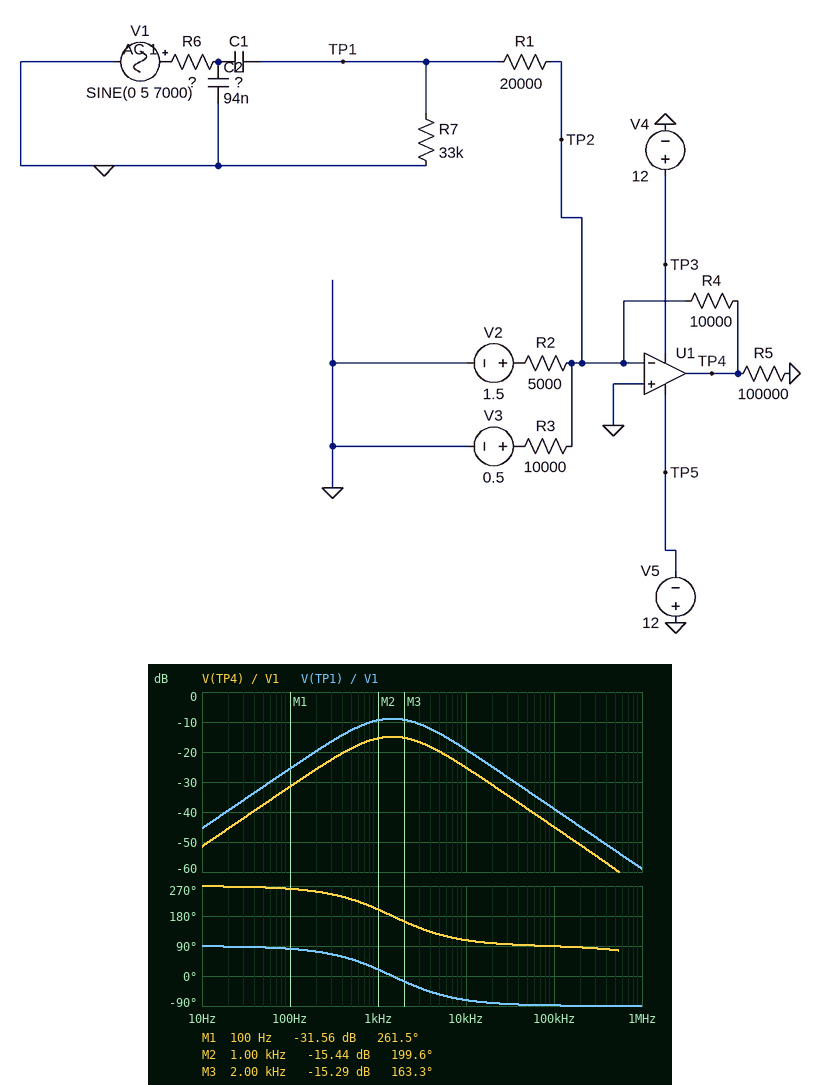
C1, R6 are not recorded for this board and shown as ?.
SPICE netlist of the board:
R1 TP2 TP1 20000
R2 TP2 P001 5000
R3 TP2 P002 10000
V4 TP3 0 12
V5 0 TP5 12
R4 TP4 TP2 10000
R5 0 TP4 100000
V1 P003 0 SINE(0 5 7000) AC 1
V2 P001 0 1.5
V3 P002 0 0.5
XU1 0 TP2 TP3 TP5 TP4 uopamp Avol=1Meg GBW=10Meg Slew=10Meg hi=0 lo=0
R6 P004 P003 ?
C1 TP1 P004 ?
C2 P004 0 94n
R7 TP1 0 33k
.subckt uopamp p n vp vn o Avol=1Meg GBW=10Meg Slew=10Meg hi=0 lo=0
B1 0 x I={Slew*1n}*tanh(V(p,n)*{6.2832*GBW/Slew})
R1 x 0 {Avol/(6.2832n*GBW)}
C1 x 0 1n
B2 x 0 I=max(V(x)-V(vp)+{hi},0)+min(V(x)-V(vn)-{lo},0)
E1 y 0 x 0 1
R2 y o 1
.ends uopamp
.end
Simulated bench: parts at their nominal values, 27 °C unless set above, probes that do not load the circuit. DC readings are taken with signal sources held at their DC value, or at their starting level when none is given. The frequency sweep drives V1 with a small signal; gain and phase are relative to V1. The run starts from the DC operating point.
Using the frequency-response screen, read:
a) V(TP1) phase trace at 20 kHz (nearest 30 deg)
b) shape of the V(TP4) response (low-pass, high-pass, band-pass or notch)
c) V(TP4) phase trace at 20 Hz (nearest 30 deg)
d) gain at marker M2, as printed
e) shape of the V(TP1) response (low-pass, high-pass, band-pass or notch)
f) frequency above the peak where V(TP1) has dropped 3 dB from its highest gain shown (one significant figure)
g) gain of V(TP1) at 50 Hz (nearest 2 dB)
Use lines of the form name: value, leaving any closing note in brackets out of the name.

V(TP1) phase trace at 20 kHz: -90 deg
shape of the V(TP4) response: band-pass
V(TP4) phase trace at 20 Hz: 270 deg
gain at marker M2, as printed: -15.44 dB
shape of the V(TP1) response: band-pass
frequency above the peak where V(TP1) has dropped 3 dB from its highest gain shown: 4 kHz
gain of V(TP1) at 50 Hz: -32 dB
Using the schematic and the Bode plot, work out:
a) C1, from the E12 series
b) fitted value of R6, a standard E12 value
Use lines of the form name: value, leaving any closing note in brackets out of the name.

C1, from the E12 series: 6.8 nF
fitted value of R6, a standard E12 value: 1.5 kΩ
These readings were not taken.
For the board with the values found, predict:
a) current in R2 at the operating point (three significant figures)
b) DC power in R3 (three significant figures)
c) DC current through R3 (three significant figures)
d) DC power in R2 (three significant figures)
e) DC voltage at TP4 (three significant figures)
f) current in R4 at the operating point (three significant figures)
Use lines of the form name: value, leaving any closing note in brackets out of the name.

current in R2 at the operating point: 300 µA
DC power in R3: 25.0 µW
DC current through R3: 50.0 µA
DC power in R2: 450 µW
DC voltage at TP4: -3.50 V
current in R4 at the operating point: 350 µA
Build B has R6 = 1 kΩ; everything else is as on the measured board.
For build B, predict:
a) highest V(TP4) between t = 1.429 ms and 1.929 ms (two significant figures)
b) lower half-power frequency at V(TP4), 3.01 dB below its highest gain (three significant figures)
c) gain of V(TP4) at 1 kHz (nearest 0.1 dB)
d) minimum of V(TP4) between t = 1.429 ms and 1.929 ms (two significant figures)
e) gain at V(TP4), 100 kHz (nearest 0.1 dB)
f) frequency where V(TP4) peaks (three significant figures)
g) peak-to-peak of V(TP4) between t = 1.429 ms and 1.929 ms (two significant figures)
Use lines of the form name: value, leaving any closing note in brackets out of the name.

highest V(TP4) between t = 1.429 ms and 1.929 ms: -2.9 V
lower half-power frequency at V(TP4), 3.01 dB below its highest gain: 719 Hz
gain of V(TP4) at 1 kHz: -14.1 dB
minimum of V(TP4) between t = 1.429 ms and 1.929 ms: -4.1 V
gain at V(TP4), 100 kHz: -41.5 dB
frequency where V(TP4) peaks: 1.78 kHz
peak-to-peak of V(TP4) between t = 1.429 ms and 1.929 ms: 1.1 V
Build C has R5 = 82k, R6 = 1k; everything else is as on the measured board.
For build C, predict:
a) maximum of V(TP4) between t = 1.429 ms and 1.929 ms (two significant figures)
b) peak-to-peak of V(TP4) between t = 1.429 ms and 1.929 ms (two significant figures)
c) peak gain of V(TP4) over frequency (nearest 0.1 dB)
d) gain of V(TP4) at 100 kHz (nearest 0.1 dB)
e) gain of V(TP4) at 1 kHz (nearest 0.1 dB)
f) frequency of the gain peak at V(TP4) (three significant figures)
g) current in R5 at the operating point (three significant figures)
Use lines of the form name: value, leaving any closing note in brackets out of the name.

maximum of V(TP4) between t = 1.429 ms and 1.929 ms: -2.9 V
peak-to-peak of V(TP4) between t = 1.429 ms and 1.929 ms: 1.1 V
peak gain of V(TP4) over frequency: -12.8 dB
gain of V(TP4) at 100 kHz: -41.5 dB
gain of V(TP4) at 1 kHz: -14.1 dB
frequency of the gain peak at V(TP4): 1.78 kHz
current in R5 at the operating point: 42.7 µA
